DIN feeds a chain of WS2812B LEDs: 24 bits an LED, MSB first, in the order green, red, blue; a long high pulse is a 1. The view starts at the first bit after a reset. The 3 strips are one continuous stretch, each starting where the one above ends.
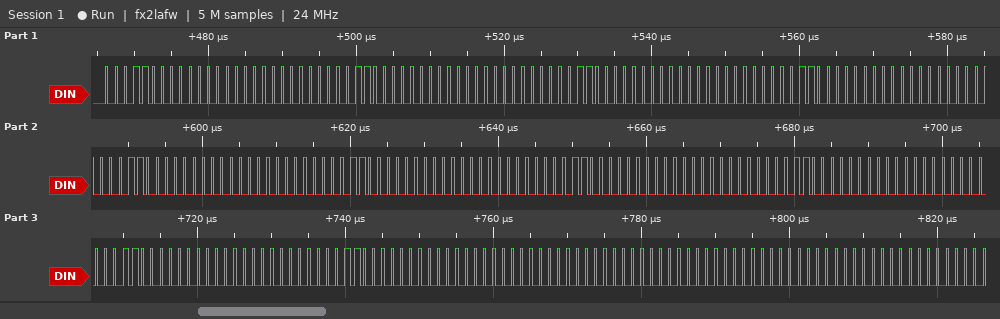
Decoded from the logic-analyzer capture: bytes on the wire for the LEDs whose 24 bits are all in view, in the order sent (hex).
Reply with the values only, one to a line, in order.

18 00 00 18 00 00 18 00 00 18 00 00 18 00 00 18 00 00 18 00 00 18 00 00 18 00 00 18 00 00 00 00 00 00 00 00
